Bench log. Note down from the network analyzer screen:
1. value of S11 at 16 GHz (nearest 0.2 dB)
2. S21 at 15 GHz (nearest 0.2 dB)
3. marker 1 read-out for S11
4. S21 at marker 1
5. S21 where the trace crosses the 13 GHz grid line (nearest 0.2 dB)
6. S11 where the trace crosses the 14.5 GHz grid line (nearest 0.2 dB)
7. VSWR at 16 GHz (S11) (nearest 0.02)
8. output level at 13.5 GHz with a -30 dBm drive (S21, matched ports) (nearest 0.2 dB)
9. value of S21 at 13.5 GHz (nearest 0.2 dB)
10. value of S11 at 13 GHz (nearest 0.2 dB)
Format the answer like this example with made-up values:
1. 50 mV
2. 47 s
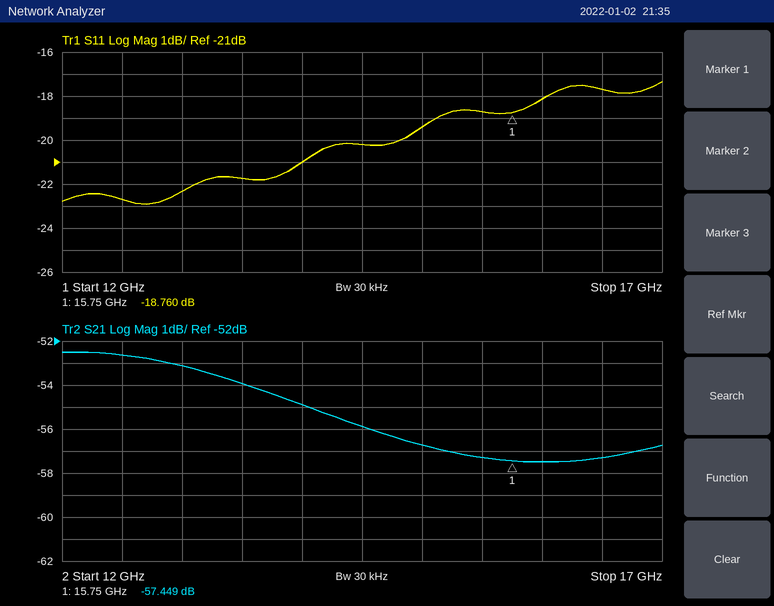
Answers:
1. -18.2 dB
2. -56.8 dB
3. -18.760 dB
4. -57.449 dB
5. -53.2 dB
6. -20.2 dB
7. 1.28
8. -84.0 dBm
9. -54.0 dB
10. -22.4 dB
